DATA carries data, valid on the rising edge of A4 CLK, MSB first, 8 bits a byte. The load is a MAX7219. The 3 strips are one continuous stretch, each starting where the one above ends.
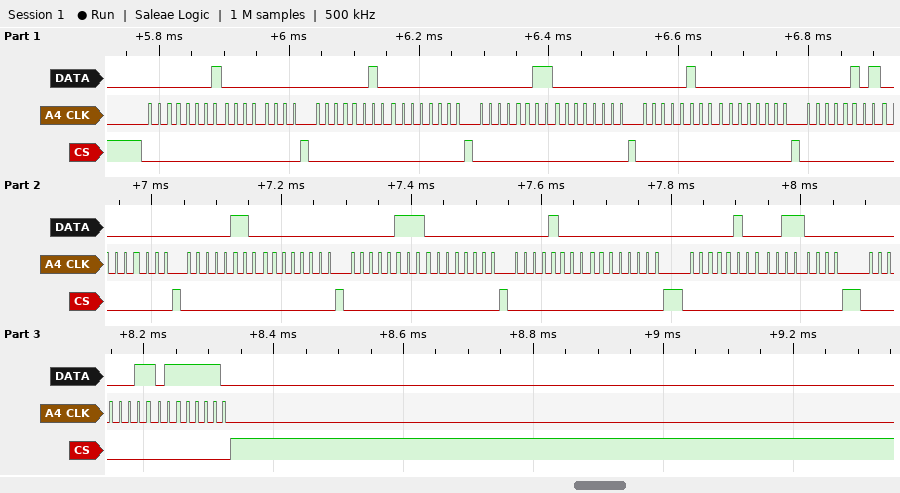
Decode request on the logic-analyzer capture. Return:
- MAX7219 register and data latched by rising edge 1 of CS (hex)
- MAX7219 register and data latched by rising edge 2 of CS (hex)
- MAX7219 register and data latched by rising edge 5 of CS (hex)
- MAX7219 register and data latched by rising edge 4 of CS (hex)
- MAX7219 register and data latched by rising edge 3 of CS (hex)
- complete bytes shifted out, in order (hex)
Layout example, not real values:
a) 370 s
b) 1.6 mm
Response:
a) register 0x1, data 0x00
b) register 0x2, data 0x00
c) register 0x5, data 0x00
d) register 0x4, data 0x00
e) register 0x3, data 0x00
f) 01 00 02 00 03 00 04 00 05 00 06 00 07 00 08 00 04 30 03 7E
